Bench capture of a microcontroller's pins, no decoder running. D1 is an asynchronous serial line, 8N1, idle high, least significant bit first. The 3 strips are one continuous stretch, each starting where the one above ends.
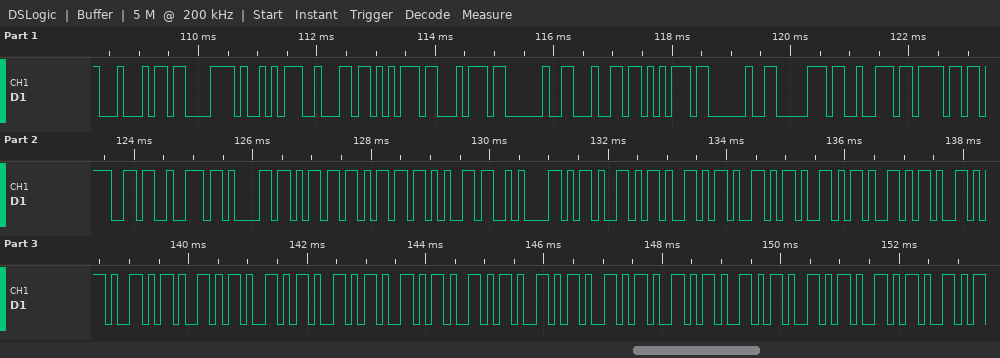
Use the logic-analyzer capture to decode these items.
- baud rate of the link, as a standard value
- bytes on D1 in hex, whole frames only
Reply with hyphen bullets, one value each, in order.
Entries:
- 9600 baud
- 44 C3 A9 62 75 74 20 64 75 20 70 72 6F 67 72 61 6D 6D 65 0A 2D 2D 2D 2D 2D 2D 2D 2D 2D 2D 2D 2D 2D 2D 2D 2D 2D 2D 2D
